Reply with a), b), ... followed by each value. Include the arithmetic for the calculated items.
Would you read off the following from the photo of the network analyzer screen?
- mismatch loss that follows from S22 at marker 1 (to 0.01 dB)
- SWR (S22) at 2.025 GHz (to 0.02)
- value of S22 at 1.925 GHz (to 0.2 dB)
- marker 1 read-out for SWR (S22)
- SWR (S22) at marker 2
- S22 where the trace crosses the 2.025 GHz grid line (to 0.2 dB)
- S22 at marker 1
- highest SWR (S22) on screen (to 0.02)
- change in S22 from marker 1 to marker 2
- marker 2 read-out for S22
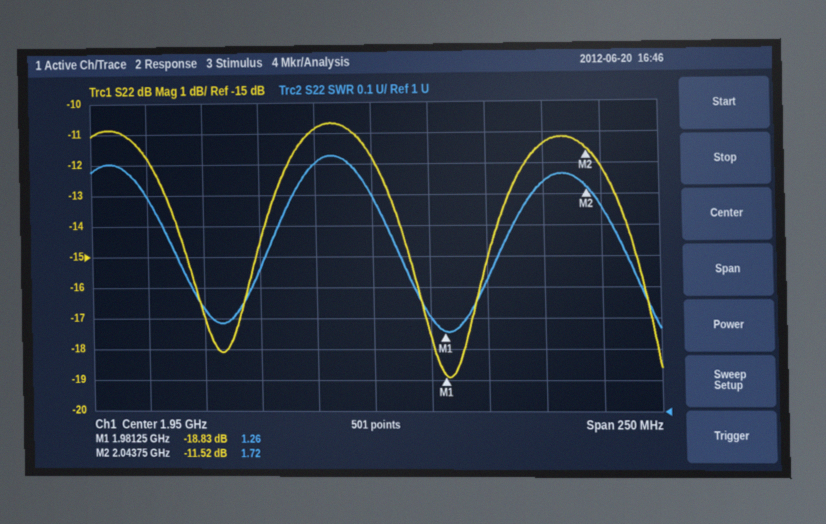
a) −10 log10(1 − 10^(-18.83/10)) ≈ 0.06 dB
b) 1.74
c) -10.8 dB
d) 1.26
e) 1.72
f) -11.4 dB
g) -18.83 dB
h) 1.82
i) -11.52 − (-18.83) = 7.31 dB
j) -11.52 dB
